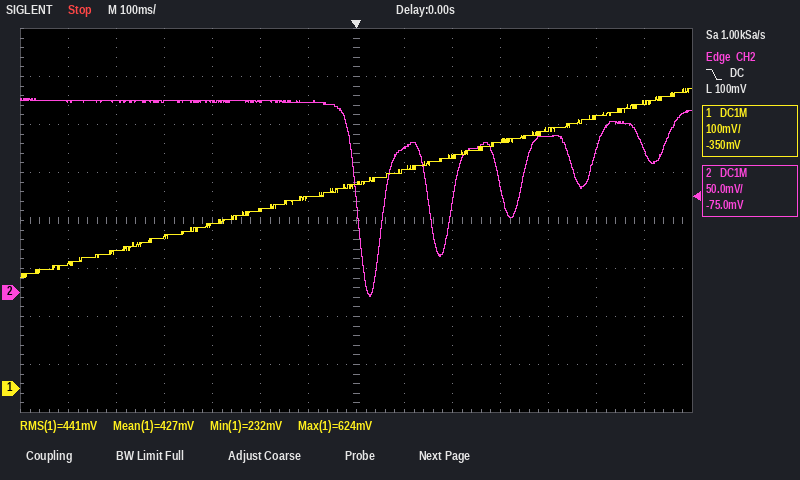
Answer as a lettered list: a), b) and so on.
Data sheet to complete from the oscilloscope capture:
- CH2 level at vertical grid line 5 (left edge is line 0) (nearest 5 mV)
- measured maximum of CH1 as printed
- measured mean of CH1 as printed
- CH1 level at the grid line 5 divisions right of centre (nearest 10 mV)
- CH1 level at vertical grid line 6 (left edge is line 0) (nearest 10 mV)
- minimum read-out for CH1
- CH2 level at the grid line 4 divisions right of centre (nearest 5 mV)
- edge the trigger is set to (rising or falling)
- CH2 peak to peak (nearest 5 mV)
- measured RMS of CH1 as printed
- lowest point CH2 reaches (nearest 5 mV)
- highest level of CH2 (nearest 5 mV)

a) 200 mV
b) 624 mV
c) 427 mV
d) 560 mV
e) 400 mV
f) 232 mV
g) 160 mV
h) falling
i) 205 mV
j) 441 mV
k) -5 mV
l) 200 mV
